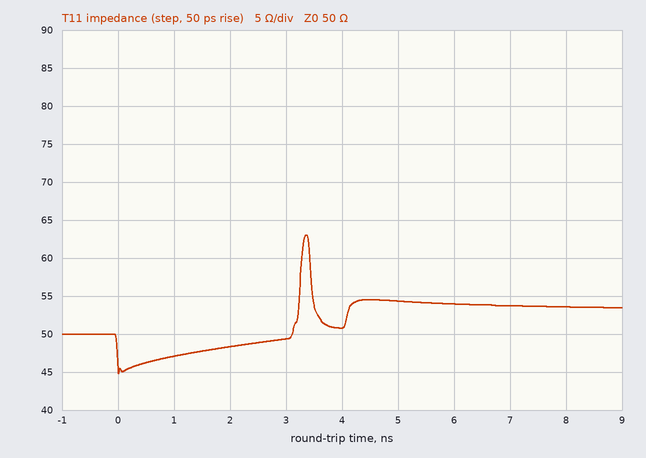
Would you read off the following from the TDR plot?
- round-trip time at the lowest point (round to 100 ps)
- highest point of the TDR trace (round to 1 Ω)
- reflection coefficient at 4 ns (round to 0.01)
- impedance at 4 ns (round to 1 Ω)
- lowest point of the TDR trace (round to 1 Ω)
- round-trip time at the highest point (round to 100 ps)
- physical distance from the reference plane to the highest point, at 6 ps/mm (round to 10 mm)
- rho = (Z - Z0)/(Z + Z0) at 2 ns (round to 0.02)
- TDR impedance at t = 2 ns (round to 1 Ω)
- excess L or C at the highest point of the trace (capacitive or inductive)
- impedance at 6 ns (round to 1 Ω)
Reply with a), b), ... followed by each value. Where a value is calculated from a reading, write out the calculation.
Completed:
a) 0.0 ns
b) 63 Ω
c) (51 − 50)/(51 + 50) ≈ +0.01
d) 51 Ω
e) 45 Ω
f) 3.4 ns
g) 3.4 ns / 2 / 6 ps/mm ≈ 283 mm, so 280 mm to the nearest 10 mm
h) (48 − 50)/(48 + 50) ≈ -0.02
i) 48 Ω
j) inductive
k) 54 Ω
